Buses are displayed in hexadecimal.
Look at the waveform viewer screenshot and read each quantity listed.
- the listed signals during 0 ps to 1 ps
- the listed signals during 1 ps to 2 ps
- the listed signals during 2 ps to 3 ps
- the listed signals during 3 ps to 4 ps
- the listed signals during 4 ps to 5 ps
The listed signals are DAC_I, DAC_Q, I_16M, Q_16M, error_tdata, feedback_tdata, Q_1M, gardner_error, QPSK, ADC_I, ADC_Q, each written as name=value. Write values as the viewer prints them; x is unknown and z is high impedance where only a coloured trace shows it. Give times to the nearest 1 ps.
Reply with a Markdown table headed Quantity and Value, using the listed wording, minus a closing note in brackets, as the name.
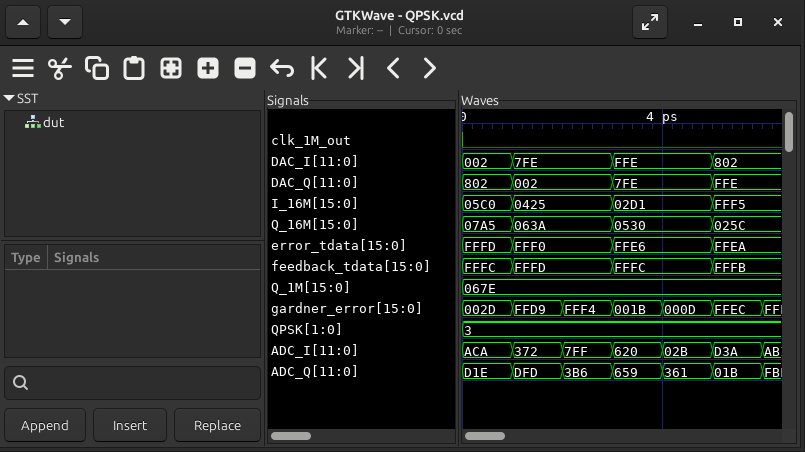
| Quantity | Value |
|---|---|
| the listed signals during 0 ps to 1 ps | DAC_I=002, DAC_Q=802, I_16M=05C0, Q_16M=07A5, error_tdata=FFFD, feedback_tdata=FFFC, Q_1M=067E, gardner_error=002D, QPSK=3, ADC_I=ACA, ADC_Q=D1E |
| the listed signals during 1 ps to 2 ps | DAC_I=7FE, DAC_Q=002, I_16M=0425, Q_16M=063A, error_tdata=FFF0, feedback_tdata=FFFD, Q_1M=067E, gardner_error=FFD9, QPSK=3, ADC_I=372, ADC_Q=DFD |
| the listed signals during 2 ps to 3 ps | DAC_I=7FE, DAC_Q=002, I_16M=0425, Q_16M=063A, error_tdata=FFF0, feedback_tdata=FFFD, Q_1M=067E, gardner_error=FFF4, QPSK=3, ADC_I=7FF, ADC_Q=3B6 |
| the listed signals during 3 ps to 4 ps | DAC_I=FFE, DAC_Q=7FE, I_16M=02D1, Q_16M=0530, error_tdata=FFE6, feedback_tdata=FFFC, Q_1M=067E, gardner_error=001B, QPSK=3, ADC_I=620, ADC_Q=659 |
| the listed signals during 4 ps to 5 ps | DAC_I=FFE, DAC_Q=7FE, I_16M=02D1, Q_16M=0530, error_tdata=FFE6, feedback_tdata=FFFC, Q_1M=067E, gardner_error=000D, QPSK=3, ADC_I=02B, ADC_Q=361 |
